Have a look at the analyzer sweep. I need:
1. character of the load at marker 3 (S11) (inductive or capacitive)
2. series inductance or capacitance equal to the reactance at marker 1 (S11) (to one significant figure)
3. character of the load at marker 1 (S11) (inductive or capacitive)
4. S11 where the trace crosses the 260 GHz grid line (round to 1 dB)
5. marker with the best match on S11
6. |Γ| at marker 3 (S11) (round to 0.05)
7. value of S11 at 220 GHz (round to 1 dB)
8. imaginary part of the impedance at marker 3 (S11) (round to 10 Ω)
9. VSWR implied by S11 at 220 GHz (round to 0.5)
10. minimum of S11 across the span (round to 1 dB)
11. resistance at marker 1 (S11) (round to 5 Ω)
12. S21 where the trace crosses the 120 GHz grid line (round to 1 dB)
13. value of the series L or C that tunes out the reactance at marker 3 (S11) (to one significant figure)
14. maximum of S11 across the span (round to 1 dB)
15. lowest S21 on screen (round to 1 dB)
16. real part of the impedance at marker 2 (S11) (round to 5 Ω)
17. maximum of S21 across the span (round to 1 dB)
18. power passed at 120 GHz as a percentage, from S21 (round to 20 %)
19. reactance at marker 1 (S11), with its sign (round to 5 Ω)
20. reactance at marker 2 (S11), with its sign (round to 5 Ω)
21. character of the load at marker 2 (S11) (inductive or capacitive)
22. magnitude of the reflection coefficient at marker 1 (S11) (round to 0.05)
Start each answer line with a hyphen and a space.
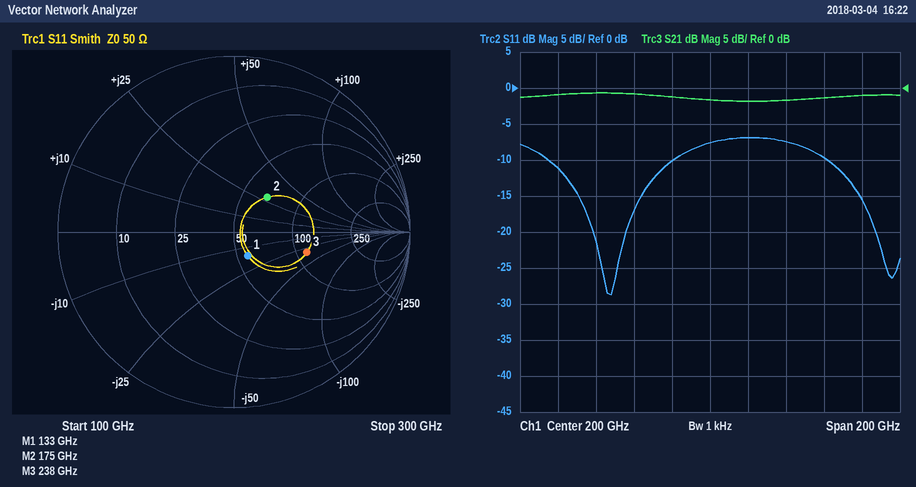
- capacitive
- 80 fF
- capacitive
- -10 dB
- marker 1
- 0.45
- -7 dB
- -30 Ω
- 2.5
- -29 dB
- 55 Ω
- -1 dB
- 20 pH
- -7 dB
- -2 dB
- 65 Ω
- -1 dB
- 80 %
- -15 Ω
- +30 Ω
- inductive
- 0.15
